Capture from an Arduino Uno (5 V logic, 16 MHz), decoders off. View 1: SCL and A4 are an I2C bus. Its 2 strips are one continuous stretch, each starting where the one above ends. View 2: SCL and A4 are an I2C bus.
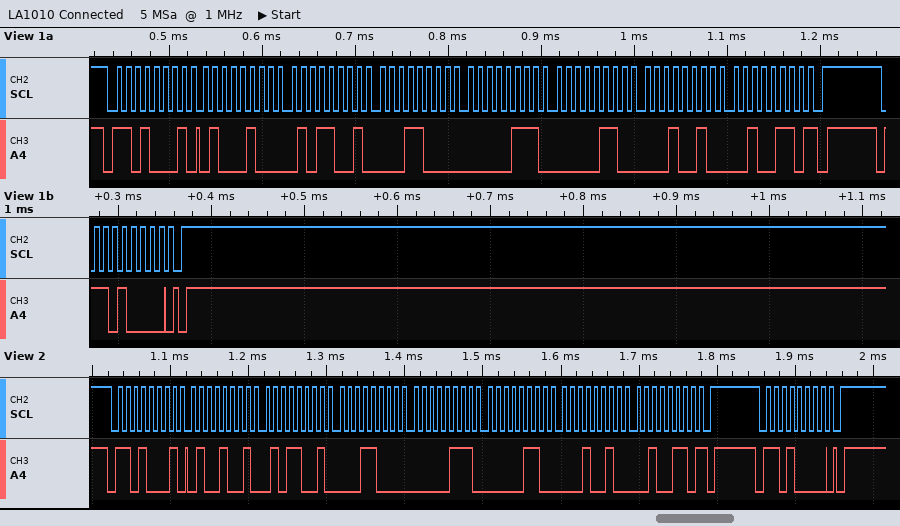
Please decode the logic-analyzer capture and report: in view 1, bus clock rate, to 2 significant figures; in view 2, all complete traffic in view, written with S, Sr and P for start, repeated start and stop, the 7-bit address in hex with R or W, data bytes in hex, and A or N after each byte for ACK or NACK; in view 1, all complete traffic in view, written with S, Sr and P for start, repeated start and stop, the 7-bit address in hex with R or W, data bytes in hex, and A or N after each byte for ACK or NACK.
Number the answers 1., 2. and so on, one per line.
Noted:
1. 100 kHz
2. S 68R A 49 A 59 A 18 A 07 A 06 A 12 A 26 N P S 68W A P
3. S 68R A 44 A 59 A 18 A 07 A 06 A 12 A 26 N P S 68W A P
